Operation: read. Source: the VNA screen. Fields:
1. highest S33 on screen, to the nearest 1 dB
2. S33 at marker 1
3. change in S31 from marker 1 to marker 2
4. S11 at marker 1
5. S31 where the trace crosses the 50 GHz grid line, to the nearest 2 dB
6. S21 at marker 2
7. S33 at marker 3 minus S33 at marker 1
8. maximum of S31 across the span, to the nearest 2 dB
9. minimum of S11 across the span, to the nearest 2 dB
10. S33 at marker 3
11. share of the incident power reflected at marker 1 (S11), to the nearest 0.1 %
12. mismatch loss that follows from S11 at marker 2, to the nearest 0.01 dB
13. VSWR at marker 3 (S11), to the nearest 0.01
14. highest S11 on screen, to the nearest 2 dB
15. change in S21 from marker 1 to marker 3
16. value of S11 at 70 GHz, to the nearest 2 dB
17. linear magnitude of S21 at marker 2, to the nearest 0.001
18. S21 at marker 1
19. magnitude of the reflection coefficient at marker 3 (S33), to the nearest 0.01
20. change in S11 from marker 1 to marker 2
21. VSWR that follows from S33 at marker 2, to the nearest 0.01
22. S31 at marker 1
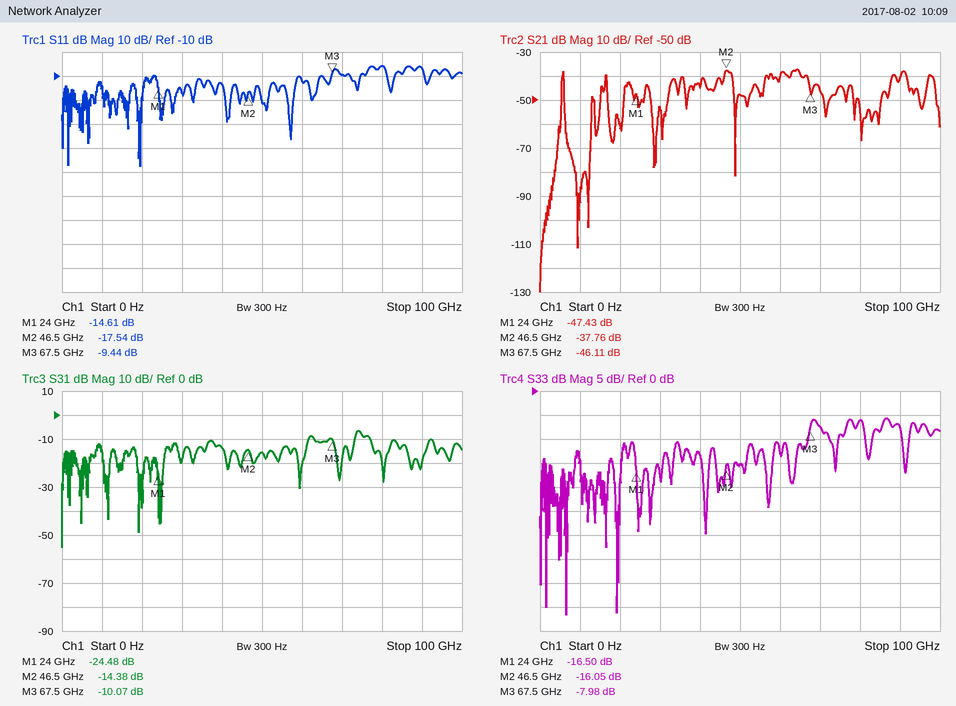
-6 dB
-16.50 dB
10.10 dB
-14.61 dB
-16 dB
-37.76 dB
8.52 dB
-6 dB
-48 dB
-7.98 dB
3.5 %
0.08 dB
2.02
-6 dB
1.32 dB
-10 dB
0.013
-47.43 dB
0.40
-2.93 dB
1.37
-24.48 dB
